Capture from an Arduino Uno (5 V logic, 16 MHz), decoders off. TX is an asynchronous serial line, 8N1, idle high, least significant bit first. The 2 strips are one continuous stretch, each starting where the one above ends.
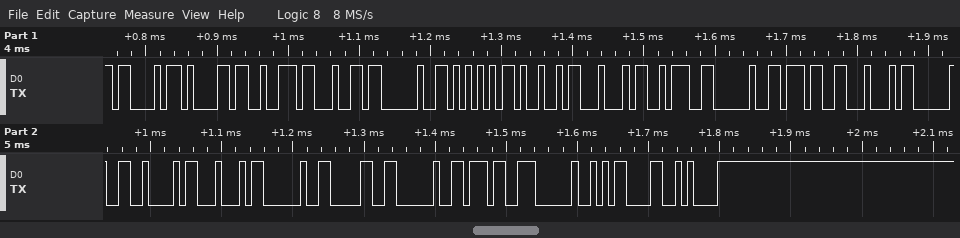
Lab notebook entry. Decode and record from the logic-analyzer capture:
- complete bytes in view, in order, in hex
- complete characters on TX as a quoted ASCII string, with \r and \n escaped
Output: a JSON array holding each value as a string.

["43 61 72 64 20 55 49 44 3A 20 37 44 20 42 44 20 30 20 37 20 0D 0A", "\"Card UID: 7D BD 0 7 \\r\\n\""]
